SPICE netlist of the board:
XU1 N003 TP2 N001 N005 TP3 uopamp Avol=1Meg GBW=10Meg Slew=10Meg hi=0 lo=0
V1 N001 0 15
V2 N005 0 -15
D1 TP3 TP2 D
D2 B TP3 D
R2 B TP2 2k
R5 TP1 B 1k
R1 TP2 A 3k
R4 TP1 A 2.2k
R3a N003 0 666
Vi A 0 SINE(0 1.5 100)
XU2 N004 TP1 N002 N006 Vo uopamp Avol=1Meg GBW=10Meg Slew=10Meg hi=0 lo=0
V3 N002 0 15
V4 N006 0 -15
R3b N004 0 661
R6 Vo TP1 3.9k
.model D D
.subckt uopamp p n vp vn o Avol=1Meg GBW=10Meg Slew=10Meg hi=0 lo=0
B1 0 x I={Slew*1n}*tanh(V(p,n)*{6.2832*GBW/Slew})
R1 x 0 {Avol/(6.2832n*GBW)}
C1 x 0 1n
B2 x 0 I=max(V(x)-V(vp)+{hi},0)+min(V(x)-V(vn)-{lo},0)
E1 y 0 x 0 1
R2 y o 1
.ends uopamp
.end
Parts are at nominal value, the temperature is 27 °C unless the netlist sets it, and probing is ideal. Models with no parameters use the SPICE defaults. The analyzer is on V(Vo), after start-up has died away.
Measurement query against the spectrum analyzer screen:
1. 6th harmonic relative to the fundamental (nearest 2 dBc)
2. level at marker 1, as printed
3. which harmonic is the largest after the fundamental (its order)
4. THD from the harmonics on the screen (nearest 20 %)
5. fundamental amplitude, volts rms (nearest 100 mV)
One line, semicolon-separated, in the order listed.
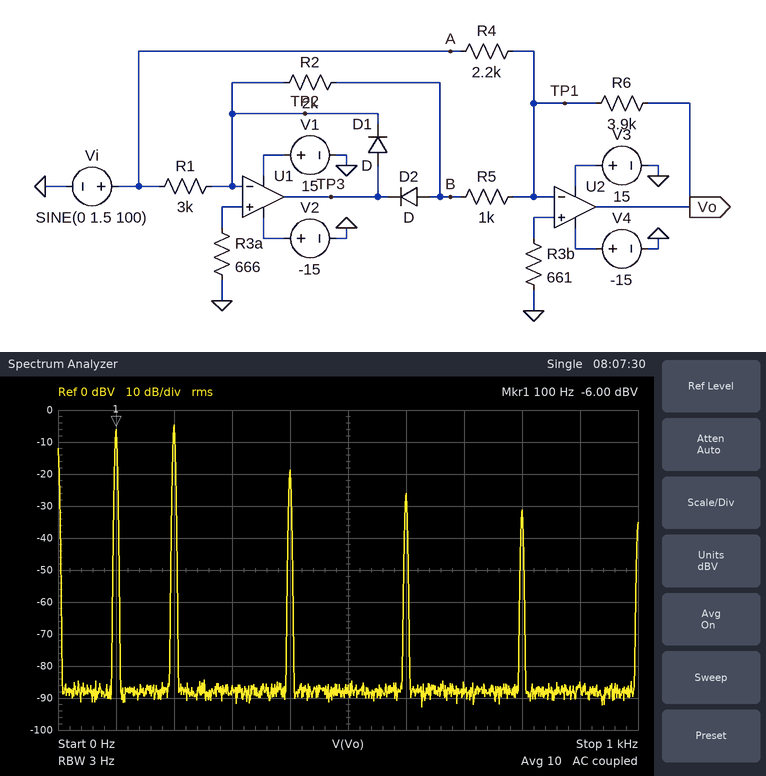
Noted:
-20 dBc; -6.00 dBV; 2; 120 %; 500 mV
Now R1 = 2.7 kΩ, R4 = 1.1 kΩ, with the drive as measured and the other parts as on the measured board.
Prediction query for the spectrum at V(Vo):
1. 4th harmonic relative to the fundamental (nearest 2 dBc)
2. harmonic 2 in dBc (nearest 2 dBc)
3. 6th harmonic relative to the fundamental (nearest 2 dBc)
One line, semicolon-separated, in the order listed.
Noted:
-24 dBc; -10 dBc; -32 dBc
